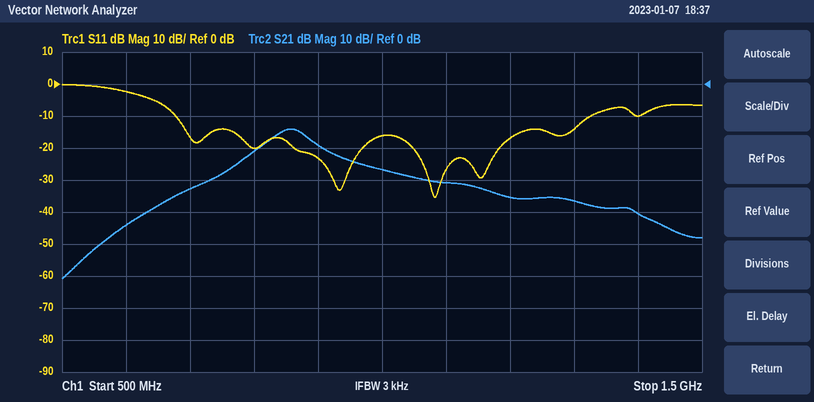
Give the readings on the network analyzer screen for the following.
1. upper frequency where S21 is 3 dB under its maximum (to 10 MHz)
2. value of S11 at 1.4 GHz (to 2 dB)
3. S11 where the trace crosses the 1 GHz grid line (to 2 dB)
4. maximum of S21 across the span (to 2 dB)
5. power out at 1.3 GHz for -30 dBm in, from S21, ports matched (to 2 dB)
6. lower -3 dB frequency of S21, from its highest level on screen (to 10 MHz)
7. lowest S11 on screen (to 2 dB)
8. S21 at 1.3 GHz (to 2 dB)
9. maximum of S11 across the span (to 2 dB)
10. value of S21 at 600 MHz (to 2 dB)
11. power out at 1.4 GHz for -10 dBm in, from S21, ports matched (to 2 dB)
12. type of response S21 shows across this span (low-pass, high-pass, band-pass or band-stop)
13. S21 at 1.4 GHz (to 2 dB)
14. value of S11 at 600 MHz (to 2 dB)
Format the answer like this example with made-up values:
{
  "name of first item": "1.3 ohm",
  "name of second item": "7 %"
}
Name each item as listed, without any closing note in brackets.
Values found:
{
  "upper frequency where S21 is 3 dB under its maximum": "890 MHz",
  "value of S11 at 1.4 GHz": "-10 dB",
  "S11 where the trace crosses the 1 GHz grid line": "-16 dB",
  "maximum of S21 across the span": "-14 dB",
  "power out at 1.3 GHz for -30 dBm in, from S21, ports matched": "-66 dBm",
  "lower -3 dB frequency of S21, from its highest level on screen": "830 MHz",
  "lowest S11 on screen": "-36 dB",
  "S21 at 1.3 GHz": "-36 dB",
  "maximum of S11 across the span": "0 dB",
  "value of S21 at 600 MHz": "-44 dB",
  "power out at 1.4 GHz for -10 dBm in, from S21, ports matched": "-50 dBm",
  "type of response S21 shows across this span": "band-pass",
  "S21 at 1.4 GHz": "-40 dB",
  "value of S11 at 600 MHz": "-2 dB"
}
